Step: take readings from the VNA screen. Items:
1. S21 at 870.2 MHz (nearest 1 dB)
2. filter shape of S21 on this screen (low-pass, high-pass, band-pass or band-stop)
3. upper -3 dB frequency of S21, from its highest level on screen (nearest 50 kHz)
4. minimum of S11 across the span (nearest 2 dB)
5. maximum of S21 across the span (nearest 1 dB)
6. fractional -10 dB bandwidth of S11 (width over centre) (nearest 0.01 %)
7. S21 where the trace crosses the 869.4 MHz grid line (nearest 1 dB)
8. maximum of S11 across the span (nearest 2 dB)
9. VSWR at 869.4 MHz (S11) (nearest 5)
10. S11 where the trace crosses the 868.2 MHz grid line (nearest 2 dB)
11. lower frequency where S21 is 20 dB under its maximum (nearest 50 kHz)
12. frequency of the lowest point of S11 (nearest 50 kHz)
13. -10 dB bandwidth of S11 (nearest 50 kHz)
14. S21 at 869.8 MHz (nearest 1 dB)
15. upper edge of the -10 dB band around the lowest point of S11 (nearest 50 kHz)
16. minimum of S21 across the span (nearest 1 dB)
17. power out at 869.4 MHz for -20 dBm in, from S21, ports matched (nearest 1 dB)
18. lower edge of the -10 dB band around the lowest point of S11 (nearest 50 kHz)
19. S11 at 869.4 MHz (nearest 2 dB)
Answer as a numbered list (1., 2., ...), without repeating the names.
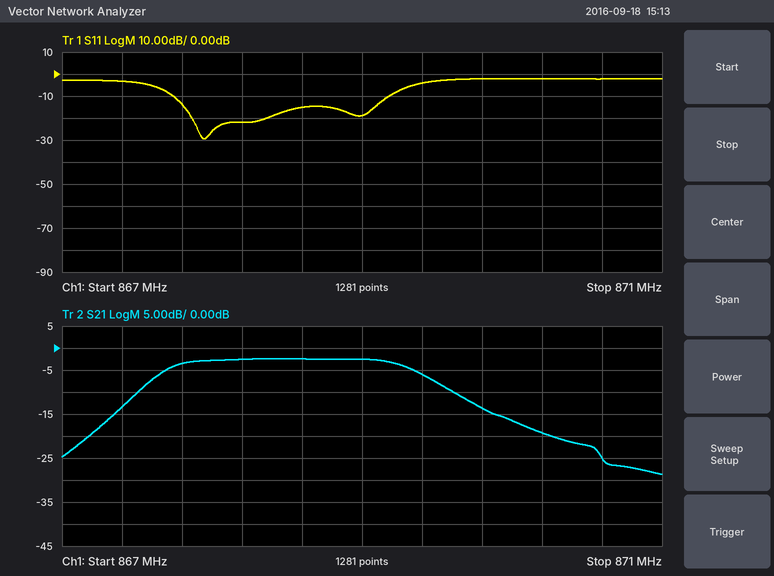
1. -19 dB
2. band-pass
3. 869.35 MHz
4. -30 dB
5. -2 dB
6. 0.17 %
7. -6 dB
8. -2 dB
9. 5
10. -22 dB
11. 867.10 MHz
12. 867.95 MHz
13. 1.45 MHz
14. -14 dB
15. 869.20 MHz
16. -29 dB
17. -26 dBm
18. 867.75 MHz
19. -4 dB
